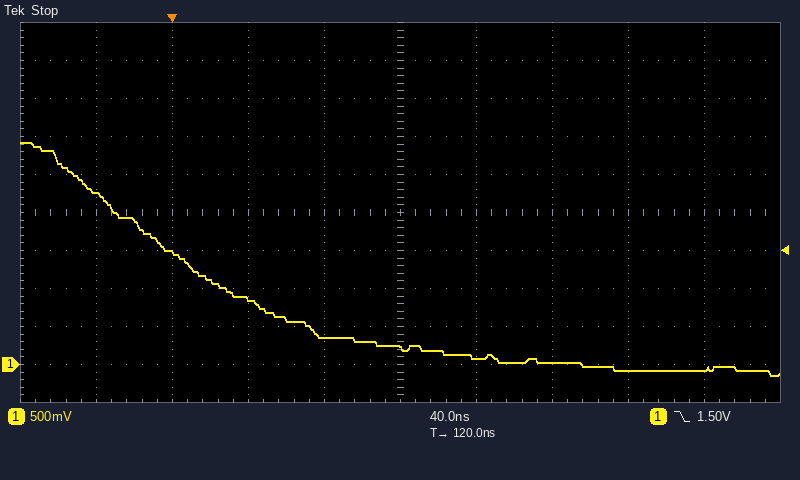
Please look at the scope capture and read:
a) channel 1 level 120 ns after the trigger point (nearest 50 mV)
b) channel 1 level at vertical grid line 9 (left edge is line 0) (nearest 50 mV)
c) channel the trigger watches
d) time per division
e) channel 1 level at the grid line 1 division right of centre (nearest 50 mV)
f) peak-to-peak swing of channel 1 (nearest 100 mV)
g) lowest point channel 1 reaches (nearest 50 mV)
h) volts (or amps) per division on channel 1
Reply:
200 mV
-50 mV
channel 1
40 ns
100 mV
3.10 V
-150 mV
500 mV
